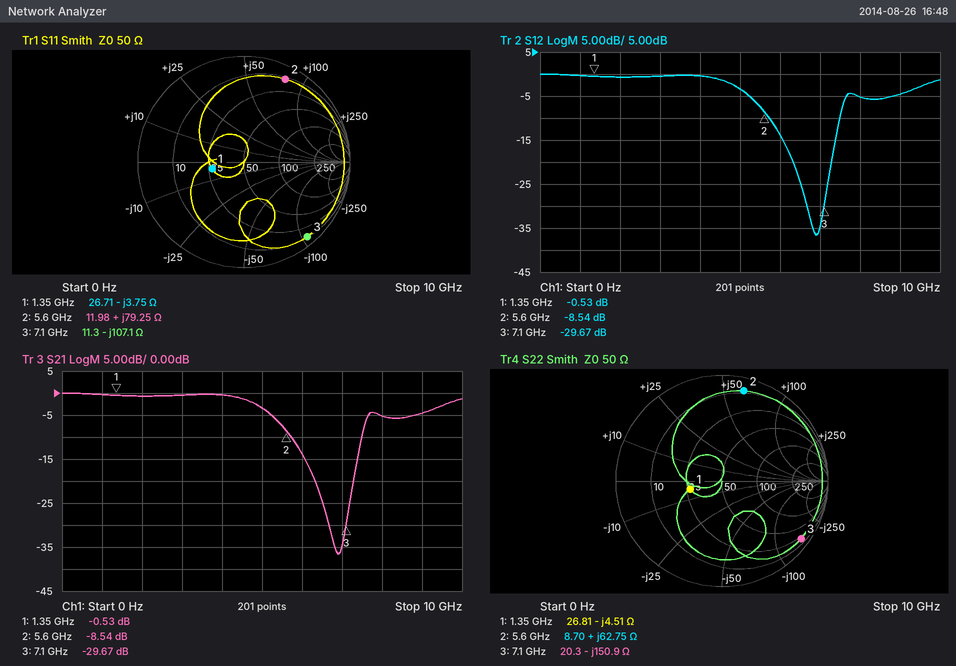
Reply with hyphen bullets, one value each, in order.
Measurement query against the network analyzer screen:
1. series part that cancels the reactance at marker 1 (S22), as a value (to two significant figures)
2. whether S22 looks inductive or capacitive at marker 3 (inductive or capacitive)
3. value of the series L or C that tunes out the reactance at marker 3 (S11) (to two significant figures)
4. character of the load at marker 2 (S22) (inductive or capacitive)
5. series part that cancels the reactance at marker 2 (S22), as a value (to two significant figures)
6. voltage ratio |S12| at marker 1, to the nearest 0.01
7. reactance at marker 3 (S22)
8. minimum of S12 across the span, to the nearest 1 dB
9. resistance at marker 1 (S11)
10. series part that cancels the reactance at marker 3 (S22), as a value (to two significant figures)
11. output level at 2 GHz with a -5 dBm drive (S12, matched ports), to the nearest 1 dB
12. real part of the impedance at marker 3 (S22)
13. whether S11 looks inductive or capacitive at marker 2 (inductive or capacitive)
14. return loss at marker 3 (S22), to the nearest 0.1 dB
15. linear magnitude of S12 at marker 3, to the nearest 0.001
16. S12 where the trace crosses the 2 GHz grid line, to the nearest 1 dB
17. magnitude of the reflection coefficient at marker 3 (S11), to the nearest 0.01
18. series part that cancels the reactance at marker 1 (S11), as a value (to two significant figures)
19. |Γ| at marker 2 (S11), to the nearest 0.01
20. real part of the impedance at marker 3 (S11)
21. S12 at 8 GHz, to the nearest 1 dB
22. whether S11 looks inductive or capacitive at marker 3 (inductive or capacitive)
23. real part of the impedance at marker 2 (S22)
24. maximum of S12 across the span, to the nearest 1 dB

- 530 pH
- capacitive
- 2.4 nH
- inductive
- 450 fF
- 0.94
- -150.9 Ω
- -37 dB
- 26.71 Ω
- 3.4 nH
- -6 dBm
- 20.3 Ω
- inductive
- 0.7 dB
- 0.033
- -1 dB
- 0.92
- 440 pH
- 0.87
- 11.3 Ω
- -5 dB
- capacitive
- 8.70 Ω
- 0 dB
